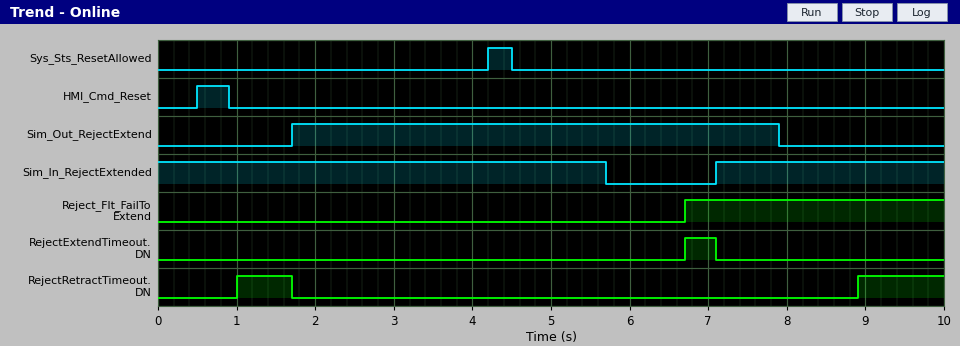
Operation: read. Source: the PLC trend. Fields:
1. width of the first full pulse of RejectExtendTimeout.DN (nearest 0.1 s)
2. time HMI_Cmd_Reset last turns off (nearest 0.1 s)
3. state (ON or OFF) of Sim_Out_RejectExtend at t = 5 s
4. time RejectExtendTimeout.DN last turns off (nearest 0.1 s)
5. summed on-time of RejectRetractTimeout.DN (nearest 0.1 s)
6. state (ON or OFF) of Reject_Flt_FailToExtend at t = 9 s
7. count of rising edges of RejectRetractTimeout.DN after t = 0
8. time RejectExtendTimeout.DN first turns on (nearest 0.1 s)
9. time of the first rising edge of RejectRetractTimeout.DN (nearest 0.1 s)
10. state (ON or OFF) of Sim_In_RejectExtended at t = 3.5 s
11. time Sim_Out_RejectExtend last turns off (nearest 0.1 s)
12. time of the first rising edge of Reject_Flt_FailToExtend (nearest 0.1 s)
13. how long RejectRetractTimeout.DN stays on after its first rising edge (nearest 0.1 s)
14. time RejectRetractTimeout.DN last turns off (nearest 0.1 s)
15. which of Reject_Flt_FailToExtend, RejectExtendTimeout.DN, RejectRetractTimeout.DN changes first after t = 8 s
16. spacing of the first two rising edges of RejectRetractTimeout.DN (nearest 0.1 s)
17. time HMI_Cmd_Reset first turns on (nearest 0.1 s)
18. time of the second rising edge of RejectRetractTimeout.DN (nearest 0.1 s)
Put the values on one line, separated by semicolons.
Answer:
0.4 s; 0.9 s; ON; 7.1 s; 1.8 s; ON; 2; 6.7 s; 1.0 s; ON; 7.9 s; 6.7 s; 0.7 s; 1.7 s; RejectRetractTimeout.DN; 7.9 s; 0.5 s; 8.9 s
